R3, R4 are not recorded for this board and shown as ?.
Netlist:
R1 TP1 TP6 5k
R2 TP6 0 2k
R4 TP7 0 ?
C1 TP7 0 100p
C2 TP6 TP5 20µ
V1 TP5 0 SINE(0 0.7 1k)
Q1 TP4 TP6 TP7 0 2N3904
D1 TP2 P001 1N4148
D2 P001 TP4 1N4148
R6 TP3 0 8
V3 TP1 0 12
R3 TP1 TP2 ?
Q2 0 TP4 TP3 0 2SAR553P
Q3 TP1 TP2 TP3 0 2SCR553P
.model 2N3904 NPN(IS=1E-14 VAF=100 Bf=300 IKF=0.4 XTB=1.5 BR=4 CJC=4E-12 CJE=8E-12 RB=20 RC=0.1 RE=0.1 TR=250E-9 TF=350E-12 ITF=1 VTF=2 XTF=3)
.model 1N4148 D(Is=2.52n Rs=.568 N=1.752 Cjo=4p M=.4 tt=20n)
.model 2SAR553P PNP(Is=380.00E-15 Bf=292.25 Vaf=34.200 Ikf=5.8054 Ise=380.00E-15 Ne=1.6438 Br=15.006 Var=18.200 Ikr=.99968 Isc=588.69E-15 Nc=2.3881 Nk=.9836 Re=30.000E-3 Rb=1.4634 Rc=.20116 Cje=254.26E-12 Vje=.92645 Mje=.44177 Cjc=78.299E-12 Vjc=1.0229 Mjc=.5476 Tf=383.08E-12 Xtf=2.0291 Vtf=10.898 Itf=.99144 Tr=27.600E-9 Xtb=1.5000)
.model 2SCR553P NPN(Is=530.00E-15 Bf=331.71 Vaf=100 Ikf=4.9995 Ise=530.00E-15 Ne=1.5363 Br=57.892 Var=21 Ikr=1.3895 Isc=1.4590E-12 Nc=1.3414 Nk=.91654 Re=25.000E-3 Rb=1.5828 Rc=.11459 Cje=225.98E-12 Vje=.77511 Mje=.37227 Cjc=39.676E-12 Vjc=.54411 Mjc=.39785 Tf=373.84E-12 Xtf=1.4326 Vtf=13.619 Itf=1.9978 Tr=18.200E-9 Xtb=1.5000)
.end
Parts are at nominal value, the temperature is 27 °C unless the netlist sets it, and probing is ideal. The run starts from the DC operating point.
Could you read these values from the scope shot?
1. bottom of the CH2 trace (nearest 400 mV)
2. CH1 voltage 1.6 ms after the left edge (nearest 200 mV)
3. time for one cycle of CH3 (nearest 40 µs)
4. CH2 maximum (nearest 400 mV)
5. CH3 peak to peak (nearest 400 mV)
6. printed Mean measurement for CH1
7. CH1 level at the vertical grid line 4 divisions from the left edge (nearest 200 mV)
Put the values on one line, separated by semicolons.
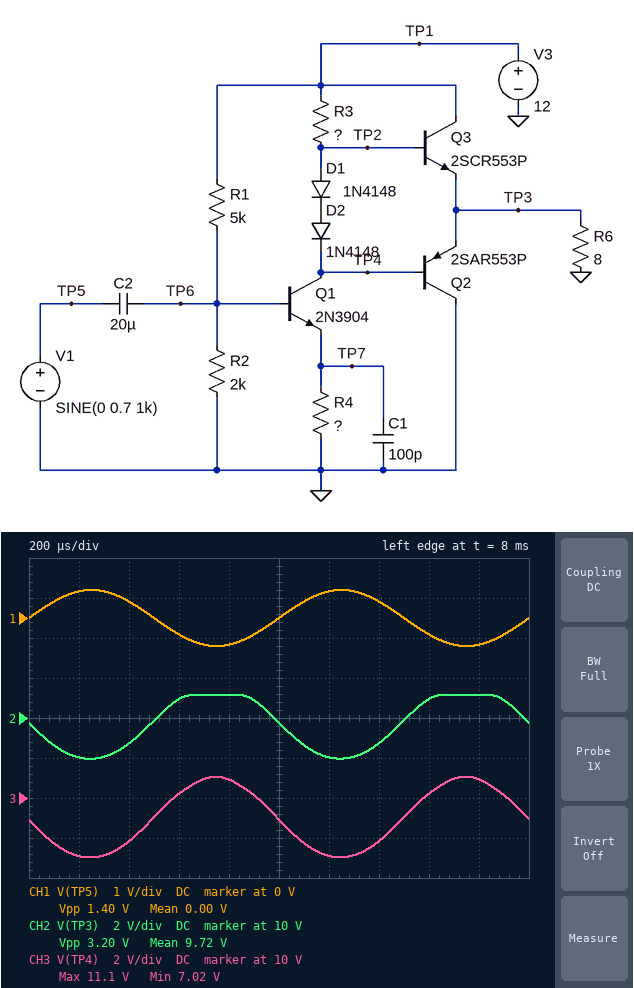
8.0 V; -400 mV; 1.00 ms; 11.2 V; 4.0 V; 0.00 V; -600 mV
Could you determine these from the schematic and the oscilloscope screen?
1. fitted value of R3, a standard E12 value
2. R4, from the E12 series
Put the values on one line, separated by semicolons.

3.3 Ω; 1.8 Ω
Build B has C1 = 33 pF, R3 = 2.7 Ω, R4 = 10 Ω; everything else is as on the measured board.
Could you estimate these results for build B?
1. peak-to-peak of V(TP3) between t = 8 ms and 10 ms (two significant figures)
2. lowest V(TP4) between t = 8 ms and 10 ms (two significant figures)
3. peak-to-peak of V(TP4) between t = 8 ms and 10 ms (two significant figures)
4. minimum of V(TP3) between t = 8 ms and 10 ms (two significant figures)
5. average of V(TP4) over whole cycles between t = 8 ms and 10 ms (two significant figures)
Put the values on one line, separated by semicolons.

710 mV; 9.2 V; 770 mV; 10 V; 9.6 V
